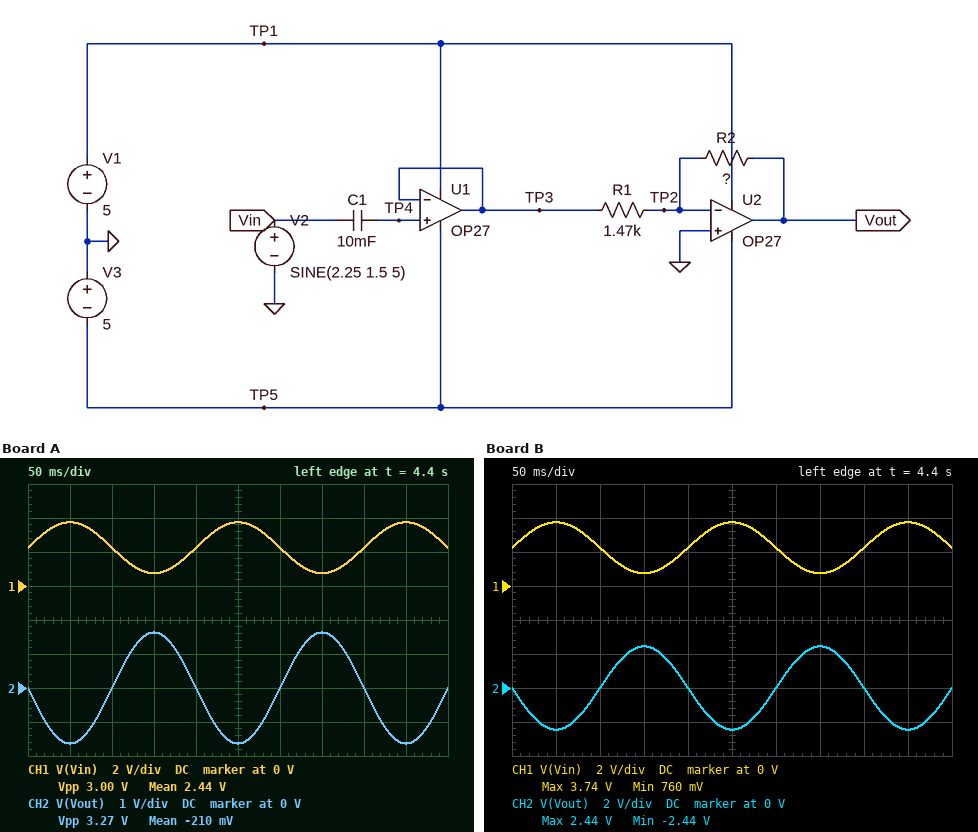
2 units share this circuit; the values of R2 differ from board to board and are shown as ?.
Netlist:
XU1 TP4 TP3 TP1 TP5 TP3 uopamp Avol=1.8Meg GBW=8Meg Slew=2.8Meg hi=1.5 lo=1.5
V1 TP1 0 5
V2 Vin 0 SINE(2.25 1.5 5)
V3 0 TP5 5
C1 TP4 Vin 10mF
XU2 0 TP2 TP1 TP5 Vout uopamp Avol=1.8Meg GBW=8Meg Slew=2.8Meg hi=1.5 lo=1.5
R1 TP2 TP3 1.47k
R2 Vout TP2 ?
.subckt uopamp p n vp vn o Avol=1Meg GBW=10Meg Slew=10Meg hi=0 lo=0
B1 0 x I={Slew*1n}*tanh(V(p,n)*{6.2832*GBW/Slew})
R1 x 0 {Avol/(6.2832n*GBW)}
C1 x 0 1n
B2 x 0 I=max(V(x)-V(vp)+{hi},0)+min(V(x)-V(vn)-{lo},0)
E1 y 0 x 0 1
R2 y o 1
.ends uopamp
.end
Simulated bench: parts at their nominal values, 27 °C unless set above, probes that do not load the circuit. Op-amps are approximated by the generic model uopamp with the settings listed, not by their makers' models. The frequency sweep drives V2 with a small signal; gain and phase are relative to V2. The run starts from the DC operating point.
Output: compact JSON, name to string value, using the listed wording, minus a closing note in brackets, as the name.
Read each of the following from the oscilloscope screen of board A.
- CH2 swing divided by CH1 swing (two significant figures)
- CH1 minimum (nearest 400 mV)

{"CH2 swing divided by CH1 swing": "1.1", "CH1 minimum": "800 mV"}
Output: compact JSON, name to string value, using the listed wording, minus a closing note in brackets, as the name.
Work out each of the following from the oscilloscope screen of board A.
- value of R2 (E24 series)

{"value of R2": "1.6 kΩ"}
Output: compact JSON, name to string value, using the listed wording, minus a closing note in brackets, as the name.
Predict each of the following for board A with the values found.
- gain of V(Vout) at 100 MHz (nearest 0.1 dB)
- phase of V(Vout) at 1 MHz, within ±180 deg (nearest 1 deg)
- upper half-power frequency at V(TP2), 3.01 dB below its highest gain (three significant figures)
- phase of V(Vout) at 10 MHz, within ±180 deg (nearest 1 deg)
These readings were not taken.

{"gain of V(Vout) at 100 MHz": "-49.6 dB", "phase of V(Vout) at 1 MHz, within ±180 deg": "158 deg", "upper half-power frequency at V(TP2), 3.01 dB below its highest gain": "14.0 MHz", "phase of V(Vout) at 10 MHz, within ±180 deg": "60 deg"}
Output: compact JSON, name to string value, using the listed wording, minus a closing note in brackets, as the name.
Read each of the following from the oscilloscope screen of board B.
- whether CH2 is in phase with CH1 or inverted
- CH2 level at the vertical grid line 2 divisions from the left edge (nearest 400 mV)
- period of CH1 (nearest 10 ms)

{"whether CH2 is in phase with CH1 or inverted": "inverted", "CH2 level at the vertical grid line 2 divisions from the left edge": "0 V", "period of CH1": "200 ms"}
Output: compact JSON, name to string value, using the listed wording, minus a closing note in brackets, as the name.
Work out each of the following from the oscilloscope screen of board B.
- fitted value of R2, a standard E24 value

{"fitted value of R2, a standard E24 value": "2.4 kΩ"}
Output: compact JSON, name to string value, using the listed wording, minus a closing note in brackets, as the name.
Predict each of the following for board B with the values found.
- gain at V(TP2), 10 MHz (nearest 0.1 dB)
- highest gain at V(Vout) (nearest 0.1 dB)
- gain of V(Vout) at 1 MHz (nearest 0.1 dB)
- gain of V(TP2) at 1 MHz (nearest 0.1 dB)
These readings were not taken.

{"gain at V(TP2), 10 MHz": "-8.6 dB", "highest gain at V(Vout)": "4.3 dB", "gain of V(Vout) at 1 MHz": "3.7 dB", "gain of V(TP2) at 1 MHz": "-14.3 dB"}
